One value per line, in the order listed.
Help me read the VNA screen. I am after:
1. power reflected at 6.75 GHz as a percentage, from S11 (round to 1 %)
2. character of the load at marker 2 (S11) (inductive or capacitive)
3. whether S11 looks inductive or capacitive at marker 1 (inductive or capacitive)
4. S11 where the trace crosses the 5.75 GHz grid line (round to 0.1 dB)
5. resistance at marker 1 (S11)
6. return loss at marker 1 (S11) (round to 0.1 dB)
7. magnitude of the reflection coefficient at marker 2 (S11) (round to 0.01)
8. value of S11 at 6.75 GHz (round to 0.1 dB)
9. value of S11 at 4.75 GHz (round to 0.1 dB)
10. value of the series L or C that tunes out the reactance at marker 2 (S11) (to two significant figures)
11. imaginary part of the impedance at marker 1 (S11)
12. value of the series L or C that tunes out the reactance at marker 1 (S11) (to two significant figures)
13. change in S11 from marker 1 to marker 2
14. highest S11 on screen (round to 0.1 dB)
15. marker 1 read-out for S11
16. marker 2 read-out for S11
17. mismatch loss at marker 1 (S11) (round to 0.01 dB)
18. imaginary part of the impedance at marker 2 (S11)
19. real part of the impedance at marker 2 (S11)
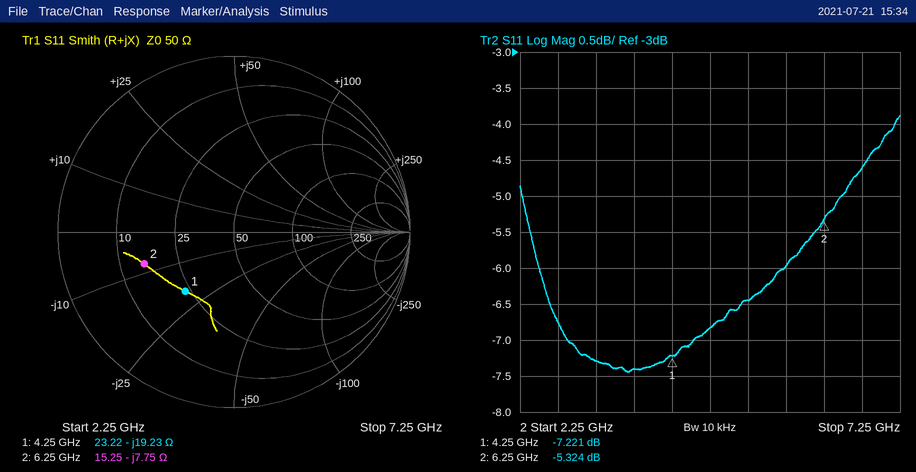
35 %
capacitive
capacitive
-6.0 dB
23.22 Ω
7.2 dB
0.54
-4.6 dB
-6.8 dB
200 pH
-19.23 Ω
720 pH
1.897 dB
-3.9 dB
-7.221 dB
-5.324 dB
0.91 dB
-7.75 Ω
15.25 Ω
